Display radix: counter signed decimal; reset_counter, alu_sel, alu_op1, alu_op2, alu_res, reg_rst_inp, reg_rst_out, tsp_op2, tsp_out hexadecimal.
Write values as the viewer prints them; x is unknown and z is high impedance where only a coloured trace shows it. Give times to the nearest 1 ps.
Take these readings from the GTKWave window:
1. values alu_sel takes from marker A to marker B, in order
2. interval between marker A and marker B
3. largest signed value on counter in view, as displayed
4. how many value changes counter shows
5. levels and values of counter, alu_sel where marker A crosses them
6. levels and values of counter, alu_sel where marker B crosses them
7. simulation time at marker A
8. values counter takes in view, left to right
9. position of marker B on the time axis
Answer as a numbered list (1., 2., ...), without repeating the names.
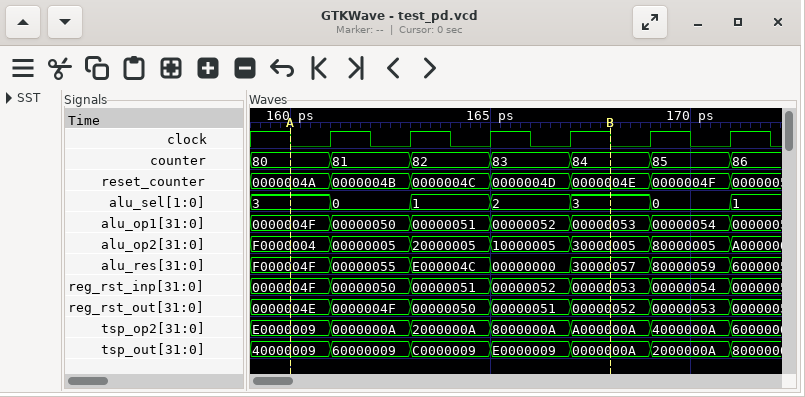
1. 3, 0, 1, 2, 3
2. 8 ps
3. 86
4. 6
5. counter=80, alu_sel=3
6. counter=84, alu_sel=3
7. 160 ps
8. 80, 81, 82, 83, 84, 85, 86
9. 168 ps
